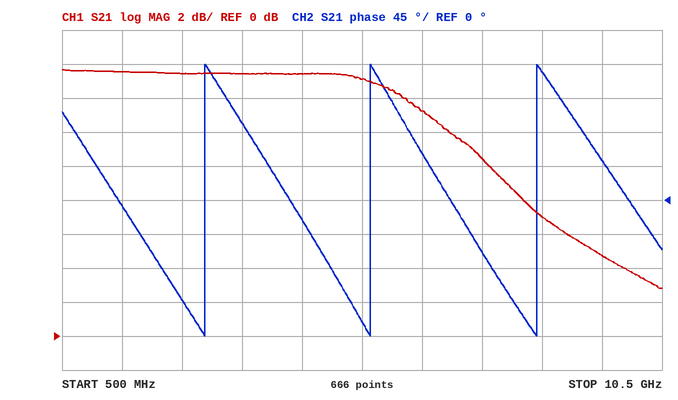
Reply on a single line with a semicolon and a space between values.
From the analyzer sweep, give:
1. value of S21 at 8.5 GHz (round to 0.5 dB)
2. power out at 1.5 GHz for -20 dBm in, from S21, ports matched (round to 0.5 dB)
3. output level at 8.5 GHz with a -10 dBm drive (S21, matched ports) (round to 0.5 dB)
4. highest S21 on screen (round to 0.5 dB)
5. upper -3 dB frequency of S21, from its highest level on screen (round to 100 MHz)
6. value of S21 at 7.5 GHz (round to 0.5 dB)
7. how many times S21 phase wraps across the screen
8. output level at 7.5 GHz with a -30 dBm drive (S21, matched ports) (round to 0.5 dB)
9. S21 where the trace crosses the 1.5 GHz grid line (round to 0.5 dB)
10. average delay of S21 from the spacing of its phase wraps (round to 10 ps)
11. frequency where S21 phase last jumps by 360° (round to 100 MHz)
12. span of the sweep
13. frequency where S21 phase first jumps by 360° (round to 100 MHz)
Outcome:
7.0 dB; -4.5 dBm; -3.0 dBm; 15.5 dB; 6.7 GHz; 10.5 dB; 3; -19.5 dBm; 15.5 dB; 360 ps; 8.4 GHz; 10 GHz; 2.9 GHz
